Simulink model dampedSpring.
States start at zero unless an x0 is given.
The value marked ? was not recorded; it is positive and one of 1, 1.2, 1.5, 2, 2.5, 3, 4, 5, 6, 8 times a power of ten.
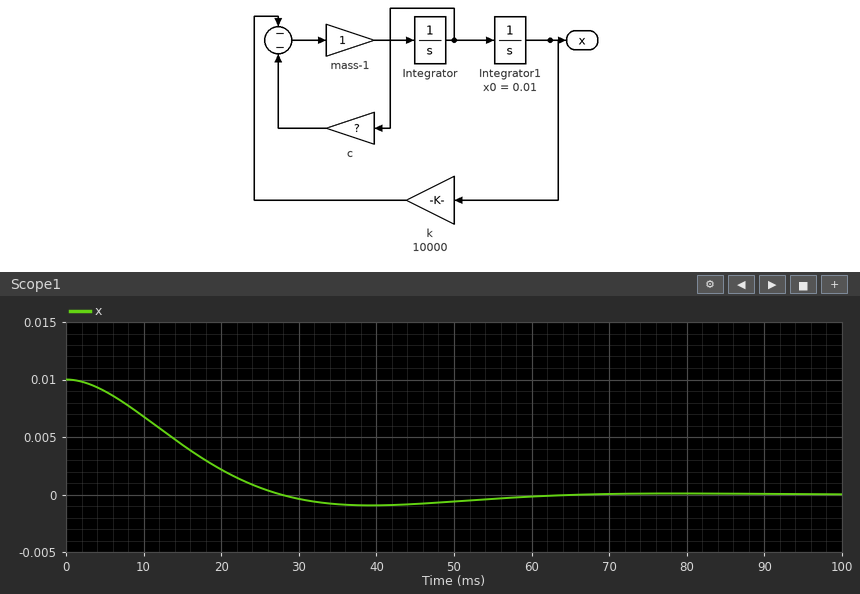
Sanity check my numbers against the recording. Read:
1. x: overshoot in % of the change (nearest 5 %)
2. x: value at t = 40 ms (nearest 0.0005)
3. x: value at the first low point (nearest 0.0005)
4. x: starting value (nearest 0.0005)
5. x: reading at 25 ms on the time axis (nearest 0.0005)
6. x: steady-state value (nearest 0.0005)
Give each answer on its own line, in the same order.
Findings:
10 %
-0.0010
-0.0010
0.0100
0.0005
0.0000
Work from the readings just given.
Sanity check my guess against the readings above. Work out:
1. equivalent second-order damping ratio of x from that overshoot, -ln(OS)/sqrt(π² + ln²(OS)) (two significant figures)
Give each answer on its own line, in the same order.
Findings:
0.59
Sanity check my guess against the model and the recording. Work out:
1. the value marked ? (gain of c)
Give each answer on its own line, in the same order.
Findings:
120
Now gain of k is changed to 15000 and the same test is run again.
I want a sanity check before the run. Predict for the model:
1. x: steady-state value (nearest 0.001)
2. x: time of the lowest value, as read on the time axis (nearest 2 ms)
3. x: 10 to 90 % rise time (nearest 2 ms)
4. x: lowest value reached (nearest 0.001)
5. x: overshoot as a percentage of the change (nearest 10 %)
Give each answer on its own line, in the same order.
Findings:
0.000
30 ms
14 ms
-0.002
20 %
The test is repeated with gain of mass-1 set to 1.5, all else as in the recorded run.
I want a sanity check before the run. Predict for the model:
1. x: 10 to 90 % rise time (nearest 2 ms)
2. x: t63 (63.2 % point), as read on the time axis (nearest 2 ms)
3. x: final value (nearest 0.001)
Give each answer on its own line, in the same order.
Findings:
18 ms
14 ms
0.000
